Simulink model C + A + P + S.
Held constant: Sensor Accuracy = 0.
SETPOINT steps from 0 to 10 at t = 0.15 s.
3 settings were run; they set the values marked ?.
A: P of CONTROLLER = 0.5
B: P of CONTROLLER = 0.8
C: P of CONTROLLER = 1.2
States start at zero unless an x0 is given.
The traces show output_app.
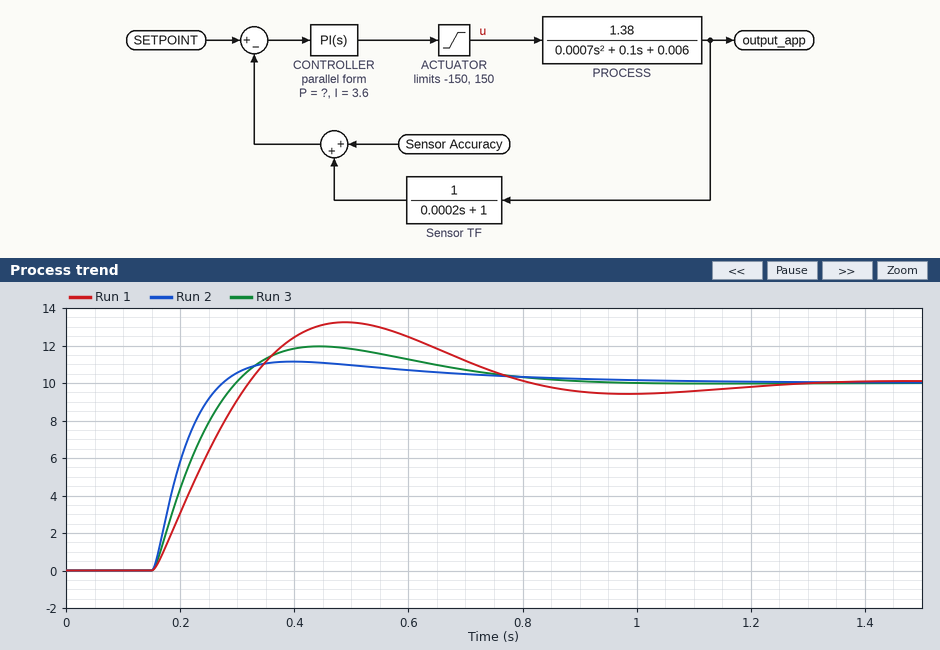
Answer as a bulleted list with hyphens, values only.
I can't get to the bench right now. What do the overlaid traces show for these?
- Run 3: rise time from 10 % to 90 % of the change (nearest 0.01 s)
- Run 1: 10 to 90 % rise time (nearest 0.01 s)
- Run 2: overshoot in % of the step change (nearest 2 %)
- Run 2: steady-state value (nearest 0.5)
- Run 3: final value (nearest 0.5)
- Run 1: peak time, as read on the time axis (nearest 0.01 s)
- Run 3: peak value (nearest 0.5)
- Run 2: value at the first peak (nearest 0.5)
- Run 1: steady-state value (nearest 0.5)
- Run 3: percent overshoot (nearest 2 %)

- 0.11 s
- 0.13 s
- 12 %
- 10.0
- 10.0
- 0.49 s
- 12.0
- 11.0
- 10.0
- 20 %
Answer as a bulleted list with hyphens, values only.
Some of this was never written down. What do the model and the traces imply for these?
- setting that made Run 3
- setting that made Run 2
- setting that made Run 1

- B
- C
- A
